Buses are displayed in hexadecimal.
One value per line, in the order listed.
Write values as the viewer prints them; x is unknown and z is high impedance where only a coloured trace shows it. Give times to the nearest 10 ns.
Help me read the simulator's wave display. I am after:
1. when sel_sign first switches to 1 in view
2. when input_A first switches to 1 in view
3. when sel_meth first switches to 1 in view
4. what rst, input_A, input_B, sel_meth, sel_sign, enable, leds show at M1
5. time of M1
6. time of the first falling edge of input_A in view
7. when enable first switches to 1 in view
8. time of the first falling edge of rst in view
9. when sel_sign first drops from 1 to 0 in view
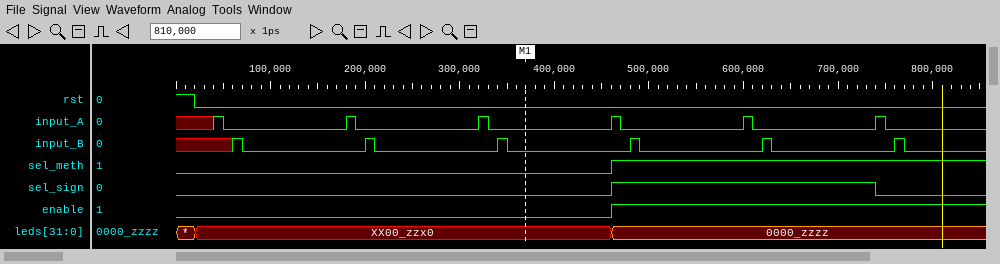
460 ns
40 ns
460 ns
rst=0, input_A=0, input_B=0, sel_meth=0, sel_sign=0, enable=0, leds=XX00_zzx0
370 ns
50 ns
460 ns
20 ns
740 ns
